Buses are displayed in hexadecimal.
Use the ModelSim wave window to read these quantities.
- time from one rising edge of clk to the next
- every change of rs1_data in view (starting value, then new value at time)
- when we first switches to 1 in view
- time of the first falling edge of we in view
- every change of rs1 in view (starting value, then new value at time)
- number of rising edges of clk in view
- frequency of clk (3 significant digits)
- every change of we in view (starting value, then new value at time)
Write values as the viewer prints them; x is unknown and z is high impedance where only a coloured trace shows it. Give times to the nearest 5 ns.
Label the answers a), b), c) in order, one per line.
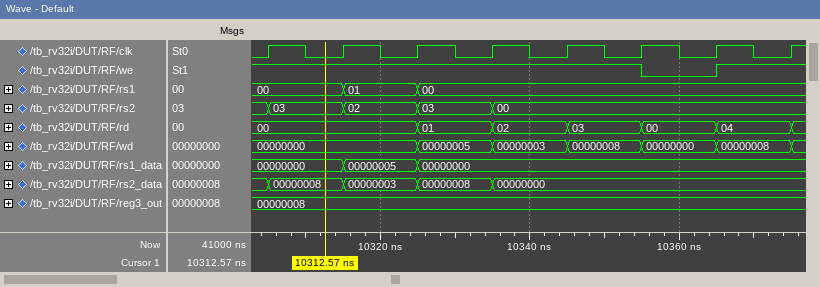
a) 10 ns
b) 00000000, 00000005 at 10315 ns, 00000000 at 10325 ns
c) 10365 ns
d) 10355 ns
e) 00, 01 at 10315 ns, 00 at 10325 ns
f) 8
g) 100 MHz
h) 1, 0 at 10355 ns, 1 at 10365 ns
